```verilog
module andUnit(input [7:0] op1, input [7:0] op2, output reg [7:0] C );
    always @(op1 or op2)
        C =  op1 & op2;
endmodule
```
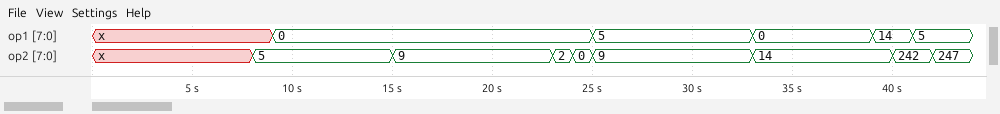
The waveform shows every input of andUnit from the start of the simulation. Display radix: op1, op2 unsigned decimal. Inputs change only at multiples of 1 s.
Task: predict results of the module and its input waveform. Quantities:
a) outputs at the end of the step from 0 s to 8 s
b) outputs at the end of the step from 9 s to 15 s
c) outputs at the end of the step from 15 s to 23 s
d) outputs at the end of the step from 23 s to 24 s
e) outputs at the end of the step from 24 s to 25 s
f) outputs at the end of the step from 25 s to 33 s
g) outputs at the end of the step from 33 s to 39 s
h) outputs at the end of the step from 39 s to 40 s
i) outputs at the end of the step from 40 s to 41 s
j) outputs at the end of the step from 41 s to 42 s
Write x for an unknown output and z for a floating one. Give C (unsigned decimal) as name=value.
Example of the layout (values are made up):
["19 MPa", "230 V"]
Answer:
["C=x", "C=0", "C=0", "C=0", "C=0", "C=1", "C=0", "C=14", "C=2", "C=0"]
